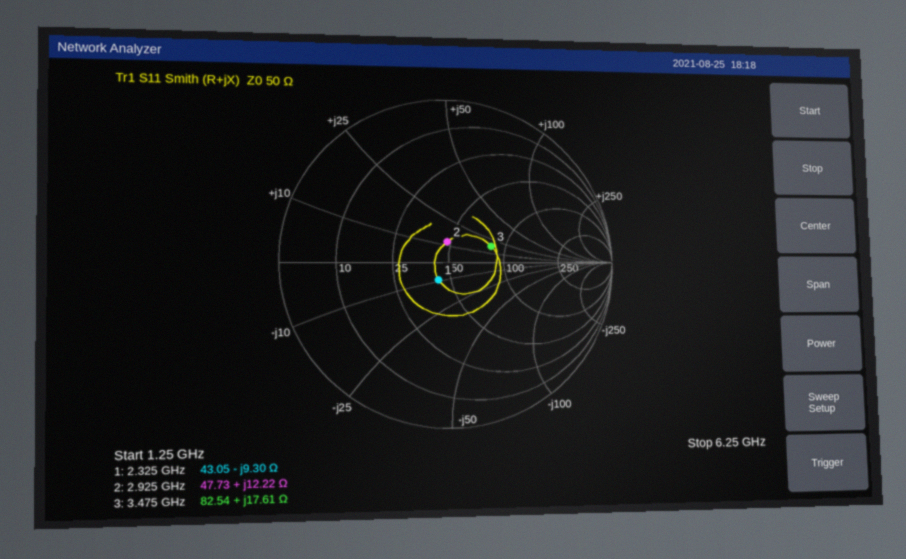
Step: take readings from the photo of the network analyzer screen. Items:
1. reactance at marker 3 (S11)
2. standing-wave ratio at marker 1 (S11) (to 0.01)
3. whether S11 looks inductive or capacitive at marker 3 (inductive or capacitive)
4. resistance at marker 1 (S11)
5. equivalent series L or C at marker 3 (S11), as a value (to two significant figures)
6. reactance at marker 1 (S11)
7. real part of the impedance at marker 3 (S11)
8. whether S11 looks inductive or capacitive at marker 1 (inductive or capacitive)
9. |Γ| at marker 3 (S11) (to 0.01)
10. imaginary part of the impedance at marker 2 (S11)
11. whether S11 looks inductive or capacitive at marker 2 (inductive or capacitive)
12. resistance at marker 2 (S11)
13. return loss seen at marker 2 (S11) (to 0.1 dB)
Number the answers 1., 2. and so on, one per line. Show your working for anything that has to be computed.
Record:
1. +17.61 Ω
2. 1.28
3. inductive
4. 43.05 Ω
5. L = 17.61 Ω/(2π × 3.475 GHz) ≈ 807 pH, so 810 pH to two significant figures
6. -9.30 Ω
7. 82.54 Ω
8. capacitive
9. 0.28
10. +12.22 Ω
11. inductive
12. 47.73 Ω
13. 18.0 dB
